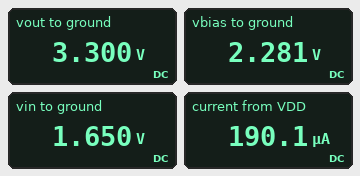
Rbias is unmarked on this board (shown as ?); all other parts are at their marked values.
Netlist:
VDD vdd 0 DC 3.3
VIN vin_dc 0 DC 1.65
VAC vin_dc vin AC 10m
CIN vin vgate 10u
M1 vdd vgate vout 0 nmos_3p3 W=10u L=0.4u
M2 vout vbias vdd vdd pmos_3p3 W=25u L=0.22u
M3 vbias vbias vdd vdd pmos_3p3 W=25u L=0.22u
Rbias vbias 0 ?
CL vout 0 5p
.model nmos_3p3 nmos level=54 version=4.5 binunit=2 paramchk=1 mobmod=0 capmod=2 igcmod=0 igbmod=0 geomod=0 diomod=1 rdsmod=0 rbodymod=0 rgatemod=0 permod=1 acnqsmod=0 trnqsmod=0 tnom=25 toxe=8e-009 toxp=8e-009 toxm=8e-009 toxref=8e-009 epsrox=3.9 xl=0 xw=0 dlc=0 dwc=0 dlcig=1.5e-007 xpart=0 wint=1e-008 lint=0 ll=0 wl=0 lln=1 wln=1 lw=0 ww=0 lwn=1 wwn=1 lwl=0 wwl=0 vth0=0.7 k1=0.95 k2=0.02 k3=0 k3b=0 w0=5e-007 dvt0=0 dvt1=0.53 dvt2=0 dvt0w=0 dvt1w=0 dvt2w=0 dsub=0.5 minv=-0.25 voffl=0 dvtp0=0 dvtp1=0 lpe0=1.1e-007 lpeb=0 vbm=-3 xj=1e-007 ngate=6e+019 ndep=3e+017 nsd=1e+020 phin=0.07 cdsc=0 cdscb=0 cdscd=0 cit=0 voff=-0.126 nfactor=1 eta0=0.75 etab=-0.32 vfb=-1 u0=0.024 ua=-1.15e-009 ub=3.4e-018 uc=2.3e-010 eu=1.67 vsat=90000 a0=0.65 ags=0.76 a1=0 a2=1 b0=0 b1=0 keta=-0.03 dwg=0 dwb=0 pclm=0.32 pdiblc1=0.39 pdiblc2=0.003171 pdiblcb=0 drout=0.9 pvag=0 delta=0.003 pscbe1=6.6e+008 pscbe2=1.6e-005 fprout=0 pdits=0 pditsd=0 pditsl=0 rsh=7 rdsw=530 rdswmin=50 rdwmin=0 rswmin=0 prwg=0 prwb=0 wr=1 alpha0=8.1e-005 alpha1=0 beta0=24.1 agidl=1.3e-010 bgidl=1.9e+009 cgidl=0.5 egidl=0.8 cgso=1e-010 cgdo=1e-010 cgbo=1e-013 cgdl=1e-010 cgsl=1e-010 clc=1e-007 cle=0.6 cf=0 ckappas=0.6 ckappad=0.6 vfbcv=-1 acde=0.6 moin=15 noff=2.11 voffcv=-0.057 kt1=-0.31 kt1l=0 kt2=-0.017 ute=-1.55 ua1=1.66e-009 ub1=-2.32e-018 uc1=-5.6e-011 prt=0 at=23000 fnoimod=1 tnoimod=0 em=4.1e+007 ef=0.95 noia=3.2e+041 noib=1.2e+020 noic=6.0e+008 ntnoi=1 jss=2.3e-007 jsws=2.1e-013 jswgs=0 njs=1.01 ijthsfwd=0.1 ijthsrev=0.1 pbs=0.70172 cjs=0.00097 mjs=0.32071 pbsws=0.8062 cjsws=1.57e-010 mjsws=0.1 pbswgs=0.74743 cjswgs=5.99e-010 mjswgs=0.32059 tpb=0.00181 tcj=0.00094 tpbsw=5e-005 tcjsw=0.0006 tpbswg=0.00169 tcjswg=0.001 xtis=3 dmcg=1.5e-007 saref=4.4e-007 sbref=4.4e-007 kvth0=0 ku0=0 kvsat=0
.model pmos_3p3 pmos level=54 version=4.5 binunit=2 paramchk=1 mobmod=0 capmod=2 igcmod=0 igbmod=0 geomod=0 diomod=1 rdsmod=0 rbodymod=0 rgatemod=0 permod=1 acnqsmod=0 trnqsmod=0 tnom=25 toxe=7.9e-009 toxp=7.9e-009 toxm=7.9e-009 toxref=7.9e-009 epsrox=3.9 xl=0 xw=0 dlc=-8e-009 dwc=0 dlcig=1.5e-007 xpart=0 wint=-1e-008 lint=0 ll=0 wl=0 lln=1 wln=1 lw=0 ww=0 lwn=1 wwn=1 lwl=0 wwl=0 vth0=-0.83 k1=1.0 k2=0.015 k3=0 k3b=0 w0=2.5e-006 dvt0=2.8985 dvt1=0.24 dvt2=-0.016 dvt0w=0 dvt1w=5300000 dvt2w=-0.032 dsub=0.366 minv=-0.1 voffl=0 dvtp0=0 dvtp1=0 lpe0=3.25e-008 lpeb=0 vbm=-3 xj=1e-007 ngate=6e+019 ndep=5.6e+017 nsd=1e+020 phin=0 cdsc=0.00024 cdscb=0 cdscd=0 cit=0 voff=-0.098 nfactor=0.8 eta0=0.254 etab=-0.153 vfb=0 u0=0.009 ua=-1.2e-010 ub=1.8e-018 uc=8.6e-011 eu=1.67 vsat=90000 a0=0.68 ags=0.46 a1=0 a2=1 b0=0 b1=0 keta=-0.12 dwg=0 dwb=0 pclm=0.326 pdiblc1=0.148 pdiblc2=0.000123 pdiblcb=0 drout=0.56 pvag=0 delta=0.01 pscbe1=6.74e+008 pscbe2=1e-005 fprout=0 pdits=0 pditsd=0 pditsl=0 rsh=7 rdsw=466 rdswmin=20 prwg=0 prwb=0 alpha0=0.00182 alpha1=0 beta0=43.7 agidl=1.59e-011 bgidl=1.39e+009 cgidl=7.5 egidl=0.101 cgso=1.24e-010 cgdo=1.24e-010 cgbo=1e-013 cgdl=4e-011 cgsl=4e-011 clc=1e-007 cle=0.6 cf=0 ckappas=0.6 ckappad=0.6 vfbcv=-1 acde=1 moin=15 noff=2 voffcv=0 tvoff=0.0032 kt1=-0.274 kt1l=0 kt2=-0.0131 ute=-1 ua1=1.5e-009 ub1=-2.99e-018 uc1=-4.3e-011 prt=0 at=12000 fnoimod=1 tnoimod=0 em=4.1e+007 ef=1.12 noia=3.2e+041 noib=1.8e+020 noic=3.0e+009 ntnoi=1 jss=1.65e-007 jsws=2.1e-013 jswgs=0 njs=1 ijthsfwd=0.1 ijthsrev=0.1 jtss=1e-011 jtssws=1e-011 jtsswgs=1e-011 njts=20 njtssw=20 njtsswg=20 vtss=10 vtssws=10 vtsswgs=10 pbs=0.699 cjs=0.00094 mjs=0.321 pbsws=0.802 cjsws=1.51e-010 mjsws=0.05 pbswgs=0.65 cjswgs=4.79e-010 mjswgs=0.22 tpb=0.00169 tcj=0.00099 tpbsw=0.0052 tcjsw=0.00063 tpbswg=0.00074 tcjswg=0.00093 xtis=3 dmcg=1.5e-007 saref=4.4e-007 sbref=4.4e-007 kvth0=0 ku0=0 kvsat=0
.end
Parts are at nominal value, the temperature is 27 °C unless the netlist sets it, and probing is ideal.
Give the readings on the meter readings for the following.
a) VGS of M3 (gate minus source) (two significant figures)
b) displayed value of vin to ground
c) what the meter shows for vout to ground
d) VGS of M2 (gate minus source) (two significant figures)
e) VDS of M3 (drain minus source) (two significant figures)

-1.0 V
1.650 V
3.300 V
-1.0 V
-1.0 V
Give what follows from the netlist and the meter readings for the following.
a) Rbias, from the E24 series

12 kΩ
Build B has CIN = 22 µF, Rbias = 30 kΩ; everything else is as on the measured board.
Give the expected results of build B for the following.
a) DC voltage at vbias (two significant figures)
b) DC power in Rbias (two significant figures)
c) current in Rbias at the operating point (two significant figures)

2.4 V
190 µW
80 µA
